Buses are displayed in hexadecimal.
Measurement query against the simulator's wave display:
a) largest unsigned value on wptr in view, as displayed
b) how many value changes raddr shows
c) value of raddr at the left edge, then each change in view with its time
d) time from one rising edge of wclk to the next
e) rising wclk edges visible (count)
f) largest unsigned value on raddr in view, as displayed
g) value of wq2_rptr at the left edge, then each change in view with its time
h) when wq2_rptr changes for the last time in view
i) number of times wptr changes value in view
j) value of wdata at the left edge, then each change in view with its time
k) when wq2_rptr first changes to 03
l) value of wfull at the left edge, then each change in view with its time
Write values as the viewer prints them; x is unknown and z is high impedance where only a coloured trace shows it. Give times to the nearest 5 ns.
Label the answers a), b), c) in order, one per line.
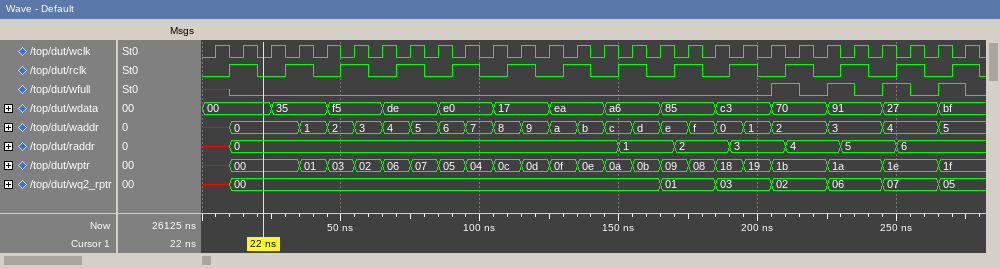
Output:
a) 1f
b) 7
c) x, 0 at 10 ns, 1 at 150 ns, 2 at 170 ns, 3 at 190 ns, 4 at 210 ns, 5 at 230 ns, 6 at 250 ns
d) 10 ns
e) 28
f) 6
g) x, 00 at 10 ns, 01 at 165 ns, 03 at 185 ns, 02 at 205 ns, 06 at 225 ns, 07 at 245 ns, 05 at 265 ns
h) 265 ns
i) 22
j) 00, 35 at 25 ns, f5 at 45 ns, de at 65 ns, e0 at 85 ns, 17 at 105 ns, ea at 125 ns, a6 at 145 ns, 85 at 165 ns, c3 at 185 ns, 70 at 205 ns, 91 at 225 ns, 27 at 245 ns, bf at 265 ns
k) 185 ns
l) x, 0 at 10 ns, 1 at 205 ns, 0 at 215 ns, 1 at 225 ns, 0 at 235 ns, 1 at 245 ns, 0 at 255 ns, 1 at 265 ns, 0 at 275 ns
